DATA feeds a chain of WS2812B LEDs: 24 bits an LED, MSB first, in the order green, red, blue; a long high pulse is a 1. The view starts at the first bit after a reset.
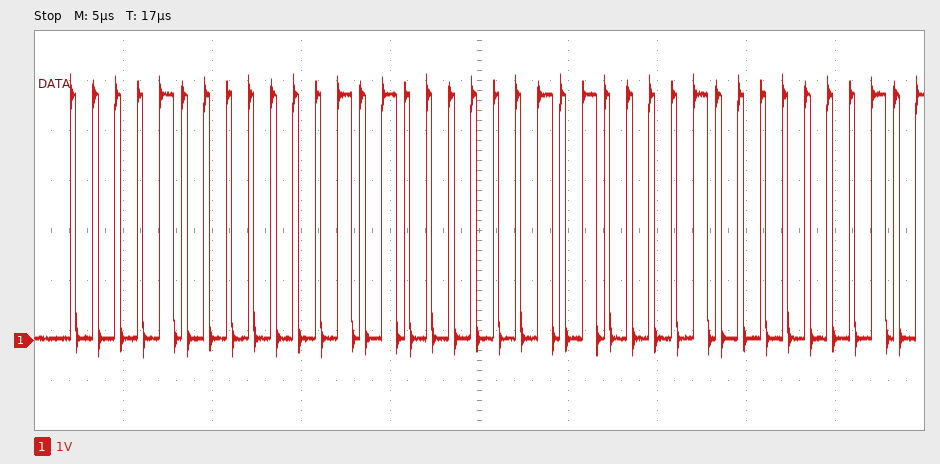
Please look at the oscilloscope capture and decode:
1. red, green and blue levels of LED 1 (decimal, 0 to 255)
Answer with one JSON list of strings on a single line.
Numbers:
["10, 8, 5"]
